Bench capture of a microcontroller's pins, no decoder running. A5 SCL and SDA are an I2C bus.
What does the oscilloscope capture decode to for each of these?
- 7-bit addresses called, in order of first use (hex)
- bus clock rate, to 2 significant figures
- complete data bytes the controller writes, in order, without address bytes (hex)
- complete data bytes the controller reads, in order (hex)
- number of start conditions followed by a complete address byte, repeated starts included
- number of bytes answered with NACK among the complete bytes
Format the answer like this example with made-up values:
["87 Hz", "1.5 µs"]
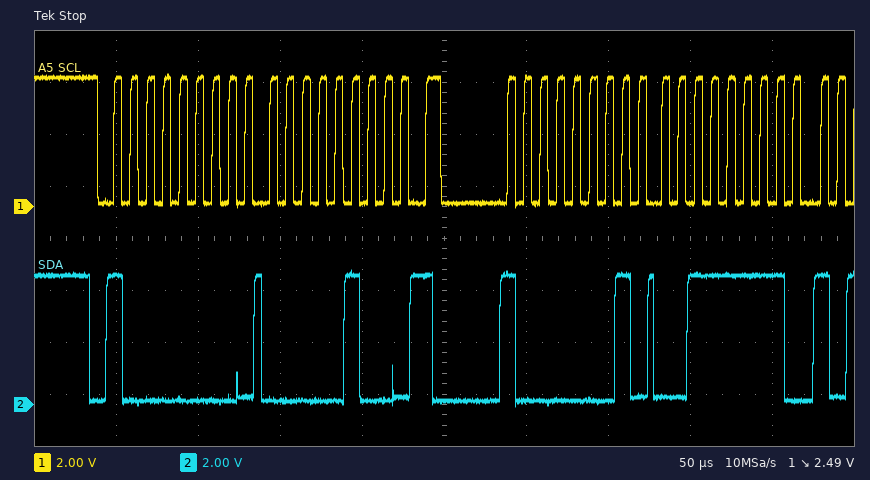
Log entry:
["0x40", "100 kHz", "04", "3F", "2", "0"]
